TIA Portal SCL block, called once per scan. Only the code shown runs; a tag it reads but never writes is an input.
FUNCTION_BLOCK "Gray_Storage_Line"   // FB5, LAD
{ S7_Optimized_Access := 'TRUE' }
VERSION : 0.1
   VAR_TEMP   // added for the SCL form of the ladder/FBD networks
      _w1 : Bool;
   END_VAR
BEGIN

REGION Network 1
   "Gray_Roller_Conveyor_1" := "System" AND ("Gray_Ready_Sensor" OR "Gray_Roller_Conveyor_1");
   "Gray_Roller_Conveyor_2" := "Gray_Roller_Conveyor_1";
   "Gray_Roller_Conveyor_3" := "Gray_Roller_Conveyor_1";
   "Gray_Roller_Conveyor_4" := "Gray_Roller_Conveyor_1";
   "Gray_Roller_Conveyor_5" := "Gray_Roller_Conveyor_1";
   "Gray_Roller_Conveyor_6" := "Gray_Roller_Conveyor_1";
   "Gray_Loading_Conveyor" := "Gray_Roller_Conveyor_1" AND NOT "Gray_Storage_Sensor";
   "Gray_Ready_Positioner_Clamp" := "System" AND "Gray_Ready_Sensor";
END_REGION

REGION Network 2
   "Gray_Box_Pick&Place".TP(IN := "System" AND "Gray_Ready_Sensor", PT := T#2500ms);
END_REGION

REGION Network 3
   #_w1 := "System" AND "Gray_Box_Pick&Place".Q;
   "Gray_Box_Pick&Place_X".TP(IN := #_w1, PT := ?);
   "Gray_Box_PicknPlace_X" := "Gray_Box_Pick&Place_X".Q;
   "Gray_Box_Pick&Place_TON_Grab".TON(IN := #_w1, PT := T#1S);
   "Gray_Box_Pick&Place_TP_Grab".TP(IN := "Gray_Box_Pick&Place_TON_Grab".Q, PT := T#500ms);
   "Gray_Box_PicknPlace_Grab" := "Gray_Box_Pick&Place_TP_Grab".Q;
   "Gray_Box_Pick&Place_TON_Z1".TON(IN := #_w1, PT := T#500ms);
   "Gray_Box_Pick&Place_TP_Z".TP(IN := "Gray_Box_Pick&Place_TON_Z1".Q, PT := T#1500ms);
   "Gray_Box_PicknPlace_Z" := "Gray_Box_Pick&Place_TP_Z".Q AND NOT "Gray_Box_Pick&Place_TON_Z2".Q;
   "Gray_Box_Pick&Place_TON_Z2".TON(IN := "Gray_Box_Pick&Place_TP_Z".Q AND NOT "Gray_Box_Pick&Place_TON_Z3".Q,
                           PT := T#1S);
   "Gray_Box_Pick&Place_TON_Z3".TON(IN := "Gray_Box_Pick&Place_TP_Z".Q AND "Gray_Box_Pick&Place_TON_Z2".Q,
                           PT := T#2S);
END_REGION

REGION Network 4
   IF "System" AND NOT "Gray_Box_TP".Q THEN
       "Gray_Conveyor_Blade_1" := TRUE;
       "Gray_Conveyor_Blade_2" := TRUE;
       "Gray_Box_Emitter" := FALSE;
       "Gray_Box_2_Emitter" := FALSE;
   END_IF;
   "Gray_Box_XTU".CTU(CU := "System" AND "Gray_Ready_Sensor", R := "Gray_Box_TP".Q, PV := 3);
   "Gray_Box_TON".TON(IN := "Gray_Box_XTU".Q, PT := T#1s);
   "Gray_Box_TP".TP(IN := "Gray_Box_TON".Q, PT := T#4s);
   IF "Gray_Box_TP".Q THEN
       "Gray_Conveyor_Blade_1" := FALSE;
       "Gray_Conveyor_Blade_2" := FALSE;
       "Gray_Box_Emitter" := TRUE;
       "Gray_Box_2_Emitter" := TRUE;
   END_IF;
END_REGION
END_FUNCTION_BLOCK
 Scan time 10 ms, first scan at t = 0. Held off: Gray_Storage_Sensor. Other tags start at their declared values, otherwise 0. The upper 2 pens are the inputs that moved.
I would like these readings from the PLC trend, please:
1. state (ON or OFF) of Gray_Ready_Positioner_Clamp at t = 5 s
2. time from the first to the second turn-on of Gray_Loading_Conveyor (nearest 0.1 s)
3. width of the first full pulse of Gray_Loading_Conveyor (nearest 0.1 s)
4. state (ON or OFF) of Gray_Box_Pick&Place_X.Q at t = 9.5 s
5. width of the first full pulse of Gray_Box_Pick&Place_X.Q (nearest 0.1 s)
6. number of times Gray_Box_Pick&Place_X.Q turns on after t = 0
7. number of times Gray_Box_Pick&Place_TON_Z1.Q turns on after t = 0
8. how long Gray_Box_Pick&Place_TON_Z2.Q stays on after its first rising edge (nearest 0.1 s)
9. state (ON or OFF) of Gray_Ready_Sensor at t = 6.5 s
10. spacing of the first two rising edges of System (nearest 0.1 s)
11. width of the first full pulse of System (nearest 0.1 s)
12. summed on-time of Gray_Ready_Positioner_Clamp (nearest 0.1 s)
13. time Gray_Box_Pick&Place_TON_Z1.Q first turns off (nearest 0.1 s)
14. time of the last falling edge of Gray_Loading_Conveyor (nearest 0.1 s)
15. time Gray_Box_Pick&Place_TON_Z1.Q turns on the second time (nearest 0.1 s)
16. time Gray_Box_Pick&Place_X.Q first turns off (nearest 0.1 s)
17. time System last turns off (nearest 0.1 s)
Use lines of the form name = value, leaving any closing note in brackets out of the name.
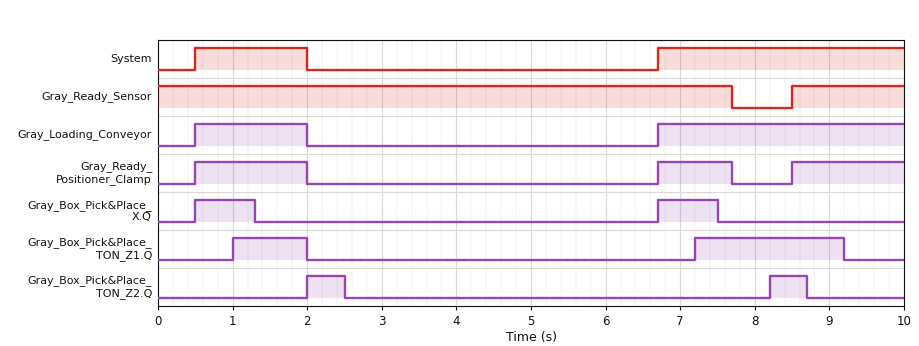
state (ON or OFF) of Gray_Ready_Positioner_Clamp at t = 5 s = OFF
time from the first to the second turn-on of Gray_Loading_Conveyor = 6.2 s
width of the first full pulse of Gray_Loading_Conveyor = 1.5 s
state (ON or OFF) of Gray_Box_Pick&Place_X.Q at t = 9.5 s = OFF
width of the first full pulse of Gray_Box_Pick&Place_X.Q = 0.8 s
number of times Gray_Box_Pick&Place_X.Q turns on after t = 0 = 2
number of times Gray_Box_Pick&Place_TON_Z1.Q turns on after t = 0 = 2
how long Gray_Box_Pick&Place_TON_Z2.Q stays on after its first rising edge = 0.5 s
state (ON or OFF) of Gray_Ready_Sensor at t = 6.5 s = ON
spacing of the first two rising edges of System = 6.2 s
width of the first full pulse of System = 1.5 s
summed on-time of Gray_Ready_Positioner_Clamp = 4.0 s
time Gray_Box_Pick&Place_TON_Z1.Q first turns off = 2.0 s
time of the last falling edge of Gray_Loading_Conveyor = 2.0 s
time Gray_Box_Pick&Place_TON_Z1.Q turns on the second time = 7.2 s
time Gray_Box_Pick&Place_X.Q first turns off = 1.3 s
time System last turns off = 2.0 s
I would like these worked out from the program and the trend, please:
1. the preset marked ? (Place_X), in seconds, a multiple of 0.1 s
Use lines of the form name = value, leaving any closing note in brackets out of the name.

the preset marked ? (Place_X), in seconds, a multiple of 0.1 s = 0.8 s
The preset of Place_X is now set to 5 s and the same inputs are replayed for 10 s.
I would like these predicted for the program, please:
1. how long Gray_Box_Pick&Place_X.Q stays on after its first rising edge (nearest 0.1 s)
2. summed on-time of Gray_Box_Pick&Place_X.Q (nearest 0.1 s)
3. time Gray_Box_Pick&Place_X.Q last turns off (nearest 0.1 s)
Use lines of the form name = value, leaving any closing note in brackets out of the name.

how long Gray_Box_Pick&Place_X.Q stays on after its first rising edge = 5.0 s
summed on-time of Gray_Box_Pick&Place_X.Q = 8.3 s
time Gray_Box_Pick&Place_X.Q last turns off = 5.5 s
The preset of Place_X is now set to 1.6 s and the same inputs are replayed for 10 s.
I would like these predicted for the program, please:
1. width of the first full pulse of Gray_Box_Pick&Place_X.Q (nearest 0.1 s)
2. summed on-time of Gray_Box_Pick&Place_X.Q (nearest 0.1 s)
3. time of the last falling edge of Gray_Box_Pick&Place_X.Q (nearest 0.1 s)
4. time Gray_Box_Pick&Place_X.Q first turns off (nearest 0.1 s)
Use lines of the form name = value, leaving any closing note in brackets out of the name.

width of the first full pulse of Gray_Box_Pick&Place_X.Q = 1.6 s
summed on-time of Gray_Box_Pick&Place_X.Q = 3.2 s
time of the last falling edge of Gray_Box_Pick&Place_X.Q = 8.3 s
time Gray_Box_Pick&Place_X.Q first turns off = 2.1 s
